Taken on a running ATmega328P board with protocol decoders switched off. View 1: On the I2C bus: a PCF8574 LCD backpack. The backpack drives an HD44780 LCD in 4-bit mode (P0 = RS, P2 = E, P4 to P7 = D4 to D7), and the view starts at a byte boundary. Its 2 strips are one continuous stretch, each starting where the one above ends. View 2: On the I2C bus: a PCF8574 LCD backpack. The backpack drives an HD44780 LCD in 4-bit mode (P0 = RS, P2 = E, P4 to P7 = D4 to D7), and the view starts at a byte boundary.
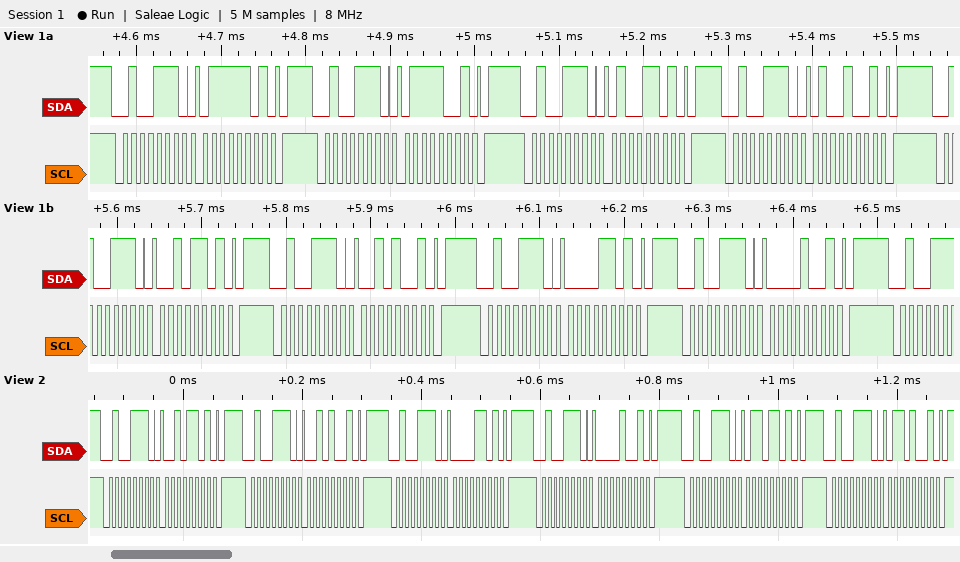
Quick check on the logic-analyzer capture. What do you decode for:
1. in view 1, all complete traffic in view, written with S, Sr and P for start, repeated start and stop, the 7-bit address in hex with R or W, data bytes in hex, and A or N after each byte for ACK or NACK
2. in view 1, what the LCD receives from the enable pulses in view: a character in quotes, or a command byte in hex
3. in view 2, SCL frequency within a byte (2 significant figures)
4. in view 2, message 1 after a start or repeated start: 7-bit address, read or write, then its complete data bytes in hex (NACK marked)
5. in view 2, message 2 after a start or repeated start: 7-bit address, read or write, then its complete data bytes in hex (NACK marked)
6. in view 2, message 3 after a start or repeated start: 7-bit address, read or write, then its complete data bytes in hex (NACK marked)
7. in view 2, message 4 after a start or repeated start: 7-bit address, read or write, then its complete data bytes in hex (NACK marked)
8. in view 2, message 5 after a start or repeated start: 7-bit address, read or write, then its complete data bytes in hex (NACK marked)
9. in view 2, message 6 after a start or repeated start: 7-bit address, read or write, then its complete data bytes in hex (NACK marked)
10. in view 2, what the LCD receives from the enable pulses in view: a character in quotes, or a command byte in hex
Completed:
S 27W A 7D A P S 27W A 79 A P S 27W A 4D A P S 27W A 49 A P S 27W A 2D A P S 27W A 29 A P S 27W A 0D A P S 27W A 09 A P
't' ' '
100 kHz
0x27 write: 2D
0x27 write: 29
0x27 write: 0D
0x27 write: 09
0x27 write: 6D
0x27 write: 69
' '
